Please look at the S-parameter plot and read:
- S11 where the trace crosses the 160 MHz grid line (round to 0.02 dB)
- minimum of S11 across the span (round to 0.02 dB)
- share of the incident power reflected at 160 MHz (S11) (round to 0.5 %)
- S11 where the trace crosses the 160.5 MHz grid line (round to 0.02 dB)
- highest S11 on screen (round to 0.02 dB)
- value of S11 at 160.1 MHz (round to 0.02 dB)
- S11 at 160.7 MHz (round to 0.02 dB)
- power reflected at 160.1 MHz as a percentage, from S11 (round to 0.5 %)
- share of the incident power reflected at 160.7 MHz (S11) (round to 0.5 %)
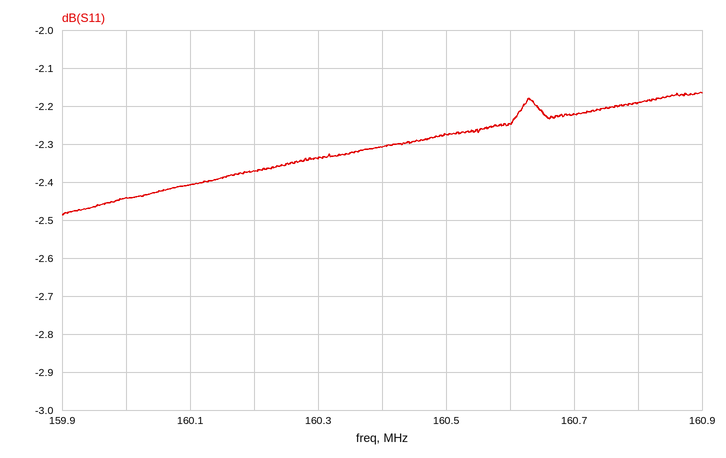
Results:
-2.44 dB
-2.48 dB
57.0 %
-2.28 dB
-2.16 dB
-2.40 dB
-2.22 dB
57.5 %
60.0 %
